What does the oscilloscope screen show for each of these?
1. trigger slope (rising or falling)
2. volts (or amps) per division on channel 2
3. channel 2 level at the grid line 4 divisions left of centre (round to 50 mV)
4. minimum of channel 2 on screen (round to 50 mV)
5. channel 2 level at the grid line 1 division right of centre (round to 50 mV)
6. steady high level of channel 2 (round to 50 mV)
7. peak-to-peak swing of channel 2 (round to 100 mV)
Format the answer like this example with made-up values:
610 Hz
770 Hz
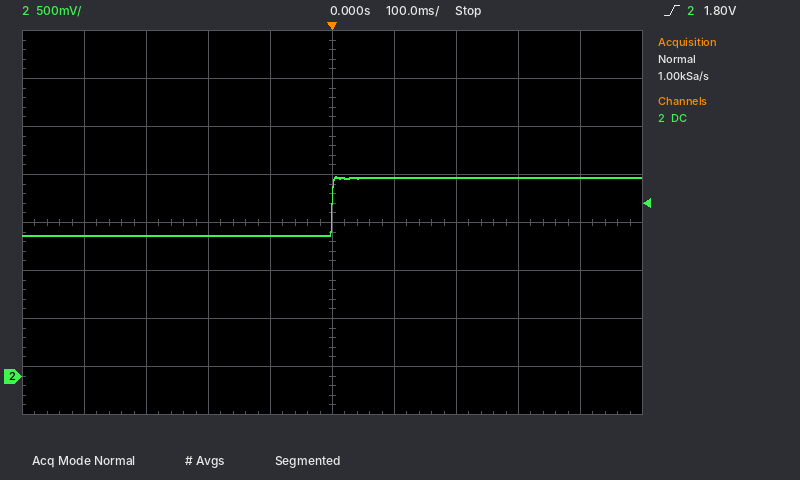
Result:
rising
500 mV
1.45 V
1.45 V
2.05 V
2.05 V
600 mV
